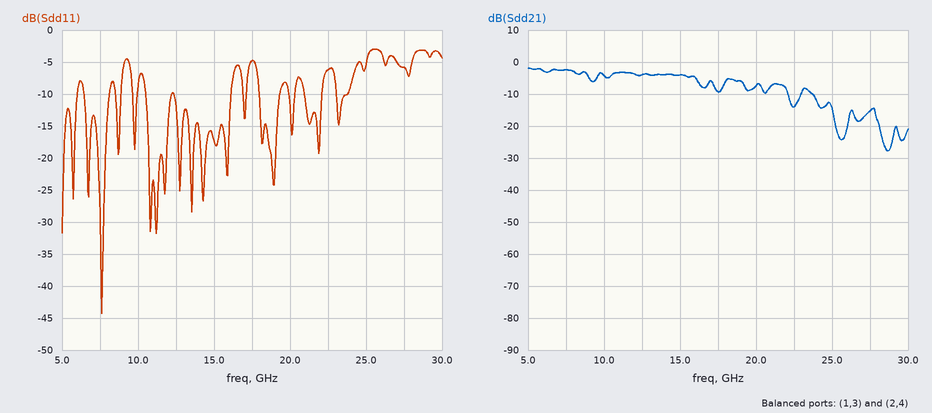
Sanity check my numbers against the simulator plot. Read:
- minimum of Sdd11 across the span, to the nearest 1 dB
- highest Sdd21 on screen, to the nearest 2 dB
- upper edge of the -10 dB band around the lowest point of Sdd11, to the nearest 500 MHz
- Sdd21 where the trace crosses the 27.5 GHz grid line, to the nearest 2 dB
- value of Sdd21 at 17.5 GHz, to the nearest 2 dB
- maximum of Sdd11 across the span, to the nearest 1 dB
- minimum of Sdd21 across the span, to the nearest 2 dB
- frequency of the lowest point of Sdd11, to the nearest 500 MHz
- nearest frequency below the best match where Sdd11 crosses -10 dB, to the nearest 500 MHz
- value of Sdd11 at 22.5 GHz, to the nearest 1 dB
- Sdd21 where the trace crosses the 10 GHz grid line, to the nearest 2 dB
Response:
-44 dB
-2 dB
8.0 GHz
-16 dB
-10 dB
-3 dB
-28 dB
7.5 GHz
6.5 GHz
-6 dB
-4 dB
